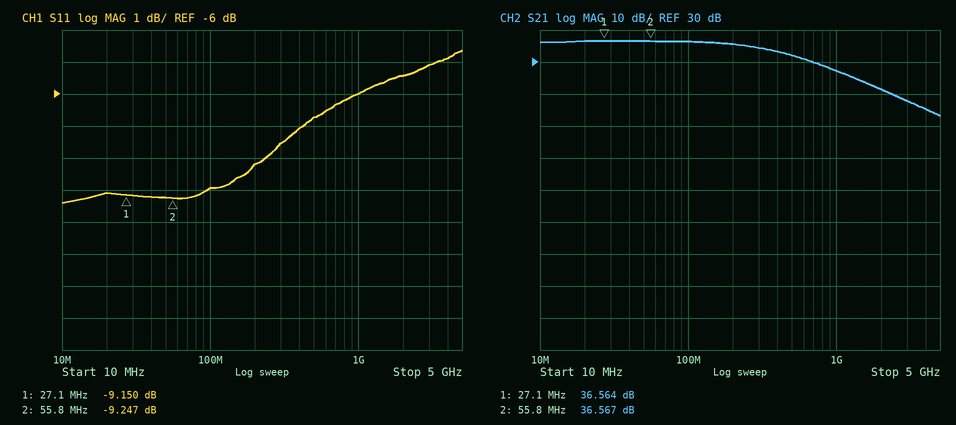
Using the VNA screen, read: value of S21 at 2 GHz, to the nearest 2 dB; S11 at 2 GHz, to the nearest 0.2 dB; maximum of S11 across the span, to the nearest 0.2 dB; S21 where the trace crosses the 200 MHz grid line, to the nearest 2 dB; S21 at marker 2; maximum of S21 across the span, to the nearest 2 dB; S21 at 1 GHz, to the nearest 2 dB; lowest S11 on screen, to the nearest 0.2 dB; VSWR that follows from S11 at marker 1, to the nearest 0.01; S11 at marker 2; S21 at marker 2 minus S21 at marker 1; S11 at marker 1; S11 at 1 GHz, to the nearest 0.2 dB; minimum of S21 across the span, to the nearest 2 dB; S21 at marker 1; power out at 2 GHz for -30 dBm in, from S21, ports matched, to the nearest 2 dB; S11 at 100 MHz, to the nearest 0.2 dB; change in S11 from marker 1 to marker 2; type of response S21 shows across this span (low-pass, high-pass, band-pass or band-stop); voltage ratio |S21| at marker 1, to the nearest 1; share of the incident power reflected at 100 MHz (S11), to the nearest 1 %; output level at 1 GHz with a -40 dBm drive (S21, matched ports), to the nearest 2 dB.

22 dB
-5.4 dB
-4.6 dB
36 dB
36.567 dB
36 dB
28 dB
-9.4 dB
2.07
-9.247 dB
0.003 dB
-9.150 dB
-6.0 dB
14 dB
36.564 dB
-8 dBm
-9.0 dB
-0.097 dB
low-pass
67
13 %
-12 dBm
